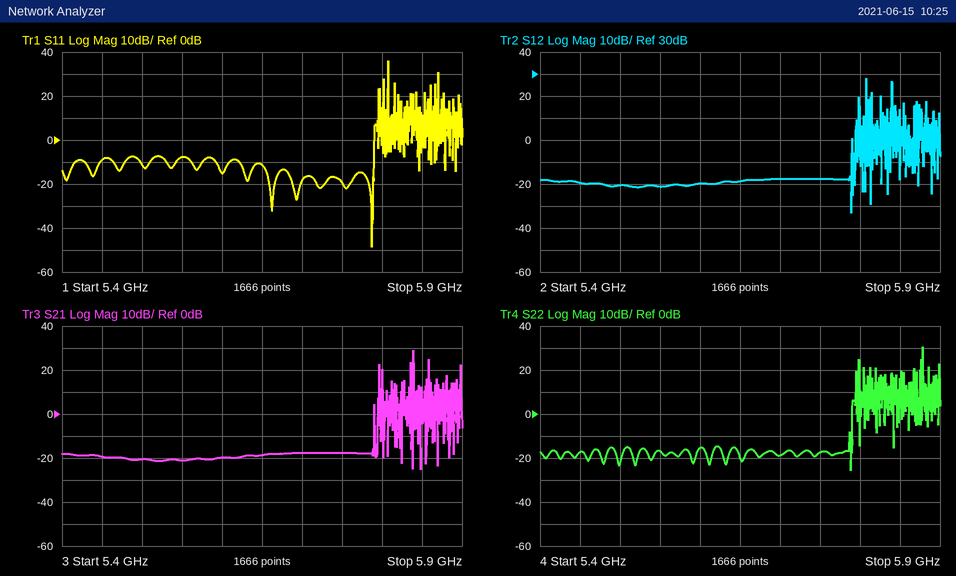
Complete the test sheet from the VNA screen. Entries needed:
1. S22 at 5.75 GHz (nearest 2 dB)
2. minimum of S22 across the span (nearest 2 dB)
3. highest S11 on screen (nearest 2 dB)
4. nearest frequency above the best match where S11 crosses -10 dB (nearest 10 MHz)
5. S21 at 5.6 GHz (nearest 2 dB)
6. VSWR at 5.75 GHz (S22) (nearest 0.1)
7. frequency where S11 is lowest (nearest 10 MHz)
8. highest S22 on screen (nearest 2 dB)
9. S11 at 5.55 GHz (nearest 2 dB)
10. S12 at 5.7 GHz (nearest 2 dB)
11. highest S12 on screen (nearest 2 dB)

-18 dB
-26 dB
36 dB
5.79 GHz
-20 dB
1.3
5.79 GHz
30 dB
-8 dB
-18 dB
28 dB
